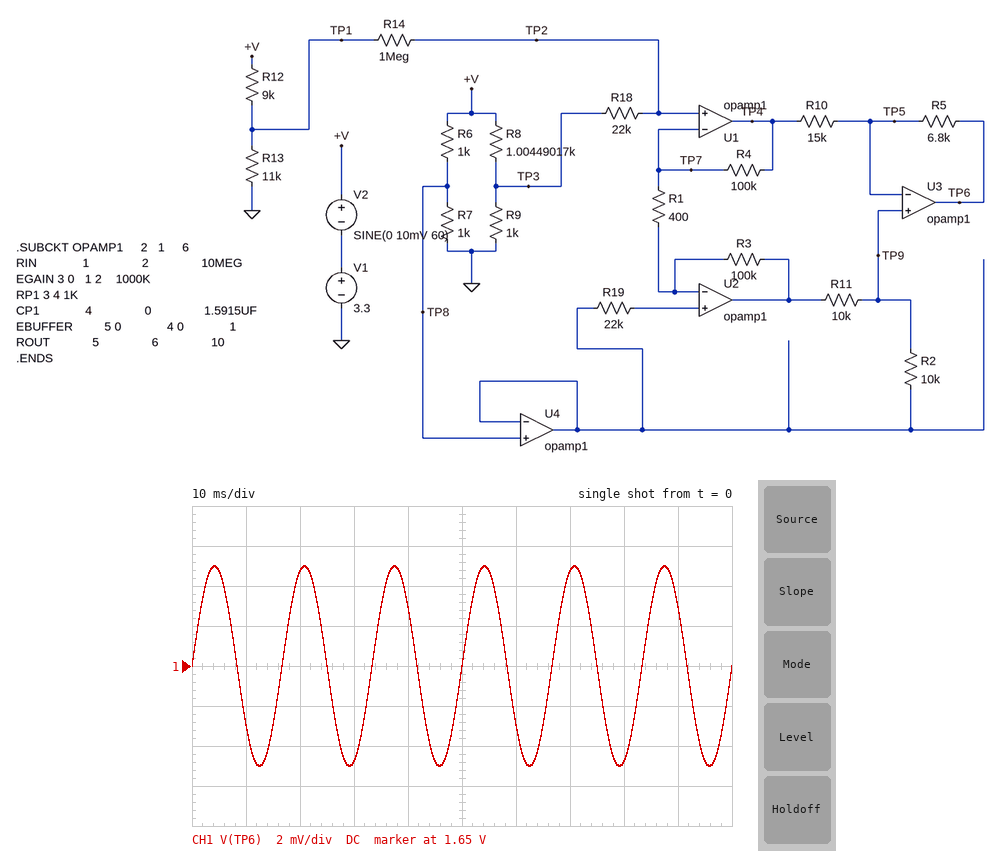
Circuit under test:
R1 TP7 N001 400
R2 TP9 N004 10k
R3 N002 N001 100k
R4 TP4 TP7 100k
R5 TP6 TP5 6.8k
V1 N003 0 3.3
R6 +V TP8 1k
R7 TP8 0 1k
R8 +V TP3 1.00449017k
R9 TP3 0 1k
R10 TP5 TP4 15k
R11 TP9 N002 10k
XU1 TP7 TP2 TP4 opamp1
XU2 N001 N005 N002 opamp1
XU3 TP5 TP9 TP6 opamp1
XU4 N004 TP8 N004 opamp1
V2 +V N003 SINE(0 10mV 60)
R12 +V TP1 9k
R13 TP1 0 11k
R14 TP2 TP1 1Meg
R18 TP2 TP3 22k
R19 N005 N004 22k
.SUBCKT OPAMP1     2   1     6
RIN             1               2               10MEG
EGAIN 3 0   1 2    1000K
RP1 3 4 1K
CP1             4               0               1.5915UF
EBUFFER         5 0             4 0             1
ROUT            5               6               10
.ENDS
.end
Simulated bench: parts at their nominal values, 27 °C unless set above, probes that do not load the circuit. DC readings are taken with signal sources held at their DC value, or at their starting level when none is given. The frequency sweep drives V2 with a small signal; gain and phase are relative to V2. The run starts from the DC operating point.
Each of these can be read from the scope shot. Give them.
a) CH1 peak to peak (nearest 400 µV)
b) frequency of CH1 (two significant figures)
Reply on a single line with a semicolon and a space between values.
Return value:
10.0 mV; 60 Hz
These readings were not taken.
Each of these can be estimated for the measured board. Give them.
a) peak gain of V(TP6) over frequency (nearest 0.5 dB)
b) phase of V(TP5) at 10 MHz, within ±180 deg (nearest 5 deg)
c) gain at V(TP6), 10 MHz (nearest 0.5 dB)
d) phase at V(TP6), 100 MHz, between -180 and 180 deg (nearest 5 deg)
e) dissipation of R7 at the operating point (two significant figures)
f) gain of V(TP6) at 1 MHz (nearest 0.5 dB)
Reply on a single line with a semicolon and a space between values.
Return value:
-6.0 dB; -10 deg; -14.0 dB; -110 deg; 2.7 mW; -13.0 dB
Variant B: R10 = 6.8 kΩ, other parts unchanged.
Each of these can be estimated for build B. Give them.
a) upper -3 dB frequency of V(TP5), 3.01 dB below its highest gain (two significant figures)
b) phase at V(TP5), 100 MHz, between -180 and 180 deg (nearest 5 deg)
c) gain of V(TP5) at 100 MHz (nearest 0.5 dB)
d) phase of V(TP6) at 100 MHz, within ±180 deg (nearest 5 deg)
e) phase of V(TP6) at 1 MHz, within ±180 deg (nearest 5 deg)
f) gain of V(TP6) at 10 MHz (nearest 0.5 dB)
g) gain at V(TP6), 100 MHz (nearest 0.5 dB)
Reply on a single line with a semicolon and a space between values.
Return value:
28 MHz; -55 deg; -13.0 dB; -115 deg; -80 deg; -40.0 dB; -65.0 dB
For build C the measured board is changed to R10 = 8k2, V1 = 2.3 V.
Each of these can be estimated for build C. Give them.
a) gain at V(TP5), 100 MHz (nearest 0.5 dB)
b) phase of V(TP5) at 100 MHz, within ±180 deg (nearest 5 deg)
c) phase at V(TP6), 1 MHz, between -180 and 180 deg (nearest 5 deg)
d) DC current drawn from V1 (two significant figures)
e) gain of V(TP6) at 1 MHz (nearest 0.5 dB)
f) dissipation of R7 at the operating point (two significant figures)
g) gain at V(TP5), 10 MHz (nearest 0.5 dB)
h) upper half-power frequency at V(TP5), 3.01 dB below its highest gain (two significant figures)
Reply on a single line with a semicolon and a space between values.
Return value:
-13.5 dB; -60 deg; -45 deg; 2.4 mA; -18.5 dB; 1.3 mW; -8.5 dB; 24 MHz
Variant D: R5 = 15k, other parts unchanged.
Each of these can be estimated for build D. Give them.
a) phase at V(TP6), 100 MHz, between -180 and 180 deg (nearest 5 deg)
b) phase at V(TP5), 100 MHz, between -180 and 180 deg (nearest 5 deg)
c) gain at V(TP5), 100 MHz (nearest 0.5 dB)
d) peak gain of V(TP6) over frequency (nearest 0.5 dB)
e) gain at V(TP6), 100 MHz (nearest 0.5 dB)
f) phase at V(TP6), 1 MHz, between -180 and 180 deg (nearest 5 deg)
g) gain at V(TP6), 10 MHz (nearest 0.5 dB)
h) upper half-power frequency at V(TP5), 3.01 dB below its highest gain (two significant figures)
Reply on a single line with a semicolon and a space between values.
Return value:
-130 deg; -55 deg; -13.0 dB; -6.0 dB; -66.0 dB; -80 deg; -40.0 dB; 28 MHz
